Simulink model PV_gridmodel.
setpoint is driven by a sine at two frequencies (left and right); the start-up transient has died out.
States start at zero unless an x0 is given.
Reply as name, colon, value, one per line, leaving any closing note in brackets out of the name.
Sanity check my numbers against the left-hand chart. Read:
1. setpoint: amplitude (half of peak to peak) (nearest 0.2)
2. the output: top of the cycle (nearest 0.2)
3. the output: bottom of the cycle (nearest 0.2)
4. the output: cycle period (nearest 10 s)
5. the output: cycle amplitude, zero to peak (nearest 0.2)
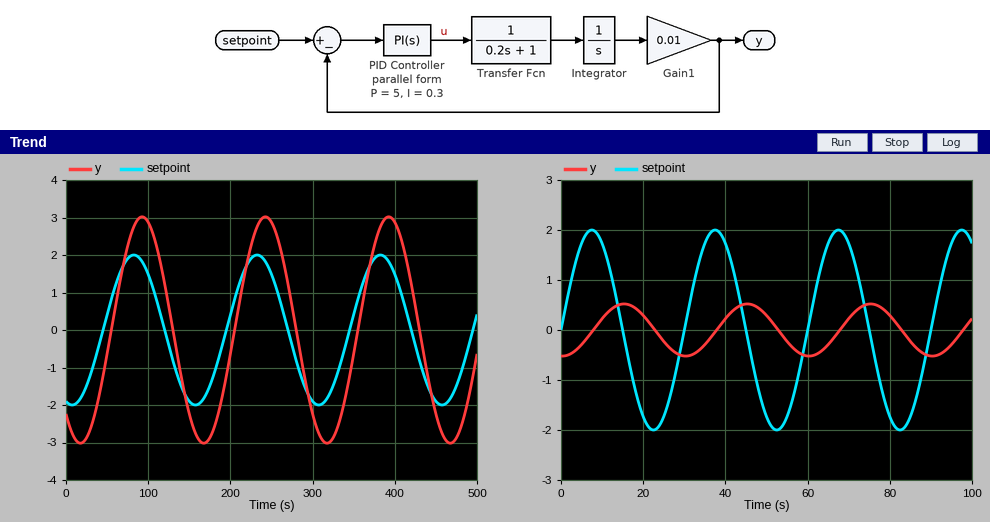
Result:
setpoint: amplitude (half of peak to peak): 2.0
the output: top of the cycle: 3.0
the output: bottom of the cycle: -3.0
the output: cycle period: 150 s
the output: cycle amplitude, zero to peak: 3.0
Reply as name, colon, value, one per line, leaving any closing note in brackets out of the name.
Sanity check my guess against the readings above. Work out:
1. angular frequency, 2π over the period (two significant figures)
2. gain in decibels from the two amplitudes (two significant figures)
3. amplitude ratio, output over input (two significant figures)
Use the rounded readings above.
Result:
angular frequency, 2π over the period: 0.042 rad/s
gain in decibels from the two amplitudes: 3.5 dB
amplitude ratio, output over input: 1.5
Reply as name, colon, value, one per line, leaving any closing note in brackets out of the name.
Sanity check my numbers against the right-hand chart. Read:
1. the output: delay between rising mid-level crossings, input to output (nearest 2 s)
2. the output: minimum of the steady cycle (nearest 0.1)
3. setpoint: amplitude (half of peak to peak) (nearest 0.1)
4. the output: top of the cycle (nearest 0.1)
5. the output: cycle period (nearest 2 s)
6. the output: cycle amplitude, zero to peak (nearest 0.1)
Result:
the output: delay between rising mid-level crossings, input to output: 8 s
the output: minimum of the steady cycle: -0.5
setpoint: amplitude (half of peak to peak): 2.0
the output: top of the cycle: 0.5
the output: cycle period: 30 s
the output: cycle amplitude, zero to peak: 0.5
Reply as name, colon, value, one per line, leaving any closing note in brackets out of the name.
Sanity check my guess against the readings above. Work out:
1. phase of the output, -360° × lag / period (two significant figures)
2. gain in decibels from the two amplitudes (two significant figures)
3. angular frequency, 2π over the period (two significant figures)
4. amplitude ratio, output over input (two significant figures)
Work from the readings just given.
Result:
phase of the output, -360° × lag / period: -96°
gain in decibels from the two amplitudes: -12 dB
angular frequency, 2π over the period: 0.21 rad/s
amplitude ratio, output over input: 0.25
